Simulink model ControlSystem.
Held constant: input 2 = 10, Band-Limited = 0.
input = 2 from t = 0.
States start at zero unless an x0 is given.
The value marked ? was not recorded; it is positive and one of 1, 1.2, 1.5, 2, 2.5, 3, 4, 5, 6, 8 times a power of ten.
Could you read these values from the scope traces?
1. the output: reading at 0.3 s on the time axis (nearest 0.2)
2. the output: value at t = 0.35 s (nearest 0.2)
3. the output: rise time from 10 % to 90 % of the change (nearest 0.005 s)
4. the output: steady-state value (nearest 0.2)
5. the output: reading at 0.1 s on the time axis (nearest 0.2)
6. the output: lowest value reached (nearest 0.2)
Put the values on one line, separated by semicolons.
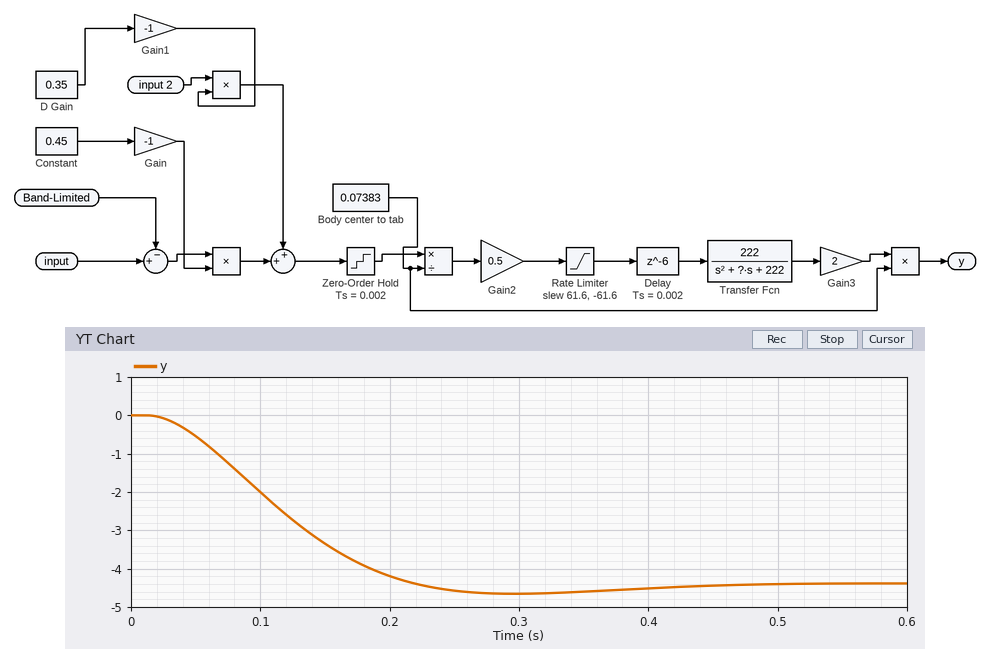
-4.6; -4.6; 0.135 s; -4.4; -2.0; -4.6
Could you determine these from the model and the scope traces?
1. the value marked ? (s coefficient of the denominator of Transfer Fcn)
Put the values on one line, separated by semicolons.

20
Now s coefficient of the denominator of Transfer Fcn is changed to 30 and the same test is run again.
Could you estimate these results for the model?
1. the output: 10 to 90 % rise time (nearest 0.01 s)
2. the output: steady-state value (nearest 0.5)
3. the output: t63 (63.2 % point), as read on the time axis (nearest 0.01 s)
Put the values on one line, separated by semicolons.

0.23 s; -4.5; 0.16 s
